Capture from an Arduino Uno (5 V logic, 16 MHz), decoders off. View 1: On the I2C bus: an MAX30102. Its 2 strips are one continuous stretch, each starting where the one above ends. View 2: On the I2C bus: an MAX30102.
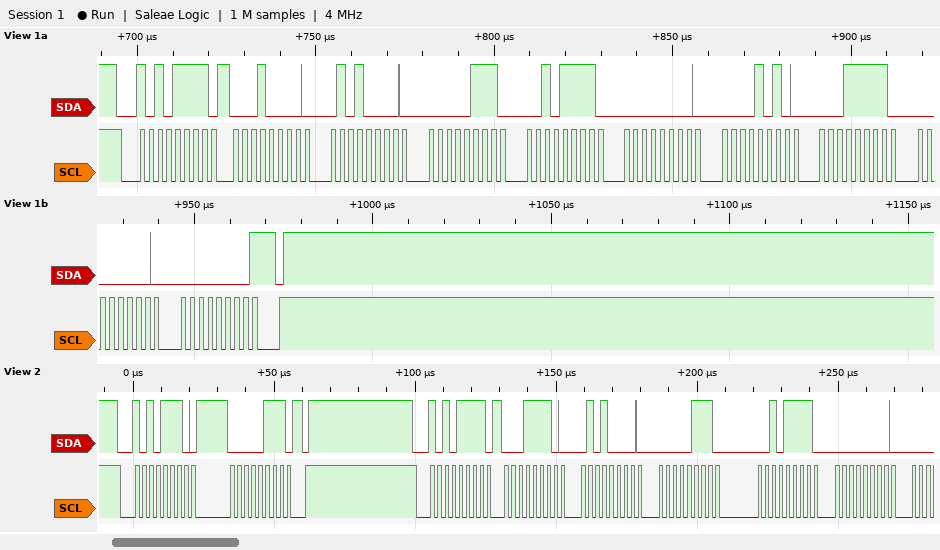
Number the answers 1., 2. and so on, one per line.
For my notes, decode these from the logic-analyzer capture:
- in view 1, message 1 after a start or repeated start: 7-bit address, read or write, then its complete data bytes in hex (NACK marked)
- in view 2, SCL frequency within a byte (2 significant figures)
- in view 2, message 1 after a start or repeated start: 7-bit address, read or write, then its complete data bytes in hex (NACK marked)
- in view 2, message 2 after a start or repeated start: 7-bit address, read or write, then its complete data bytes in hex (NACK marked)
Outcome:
1. 0x57 read: 10 50 07 2F 00 0A 1F 00 00 NACK
2. 400 kHz
3. 0x57 write: 07
4. 0x57 read: 1E 50 07 2F 00
